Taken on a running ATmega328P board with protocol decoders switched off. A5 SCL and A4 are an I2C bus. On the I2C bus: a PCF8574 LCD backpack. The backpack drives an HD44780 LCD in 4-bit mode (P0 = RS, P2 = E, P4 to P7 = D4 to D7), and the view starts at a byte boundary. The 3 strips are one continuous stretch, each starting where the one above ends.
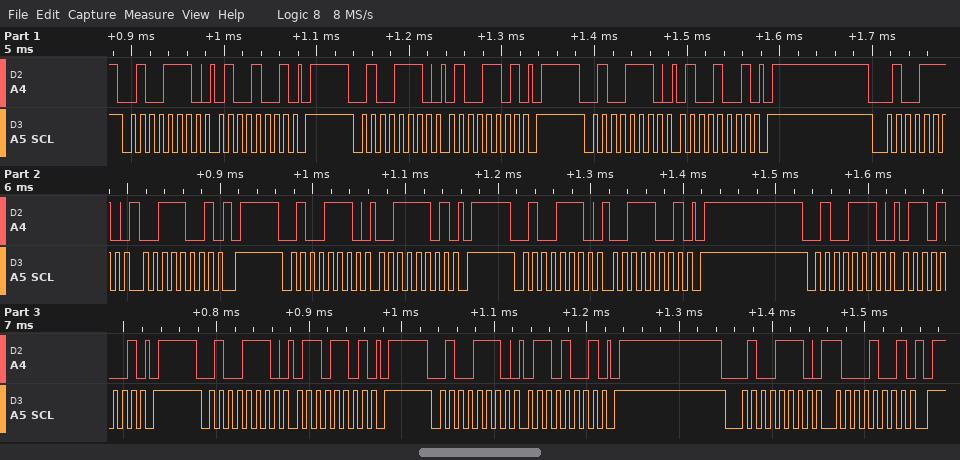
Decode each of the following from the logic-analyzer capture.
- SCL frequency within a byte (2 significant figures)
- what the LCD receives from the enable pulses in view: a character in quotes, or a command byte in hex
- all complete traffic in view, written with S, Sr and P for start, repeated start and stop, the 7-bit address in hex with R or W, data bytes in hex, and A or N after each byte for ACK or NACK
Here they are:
100 kHz
'C'
S 27W A 49 A P S 27W A 4D A P S 27W A 49 A P S 27W A 39 A P S 27W A 3D A P S 27W A 39 A P S 27W A 69 A P S 27W A 6D A P S 27W A 69 A P S 27W A 89 A P
